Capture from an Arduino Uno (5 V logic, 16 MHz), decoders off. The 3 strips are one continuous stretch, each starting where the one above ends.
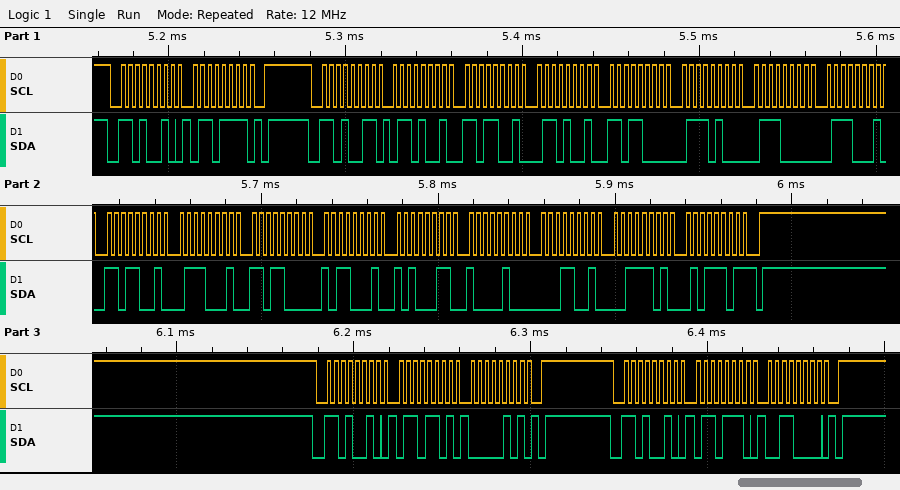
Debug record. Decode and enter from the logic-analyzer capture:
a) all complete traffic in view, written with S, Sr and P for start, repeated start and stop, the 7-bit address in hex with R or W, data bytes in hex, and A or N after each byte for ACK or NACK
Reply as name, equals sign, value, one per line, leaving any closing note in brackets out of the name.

all complete traffic in view, written with S, Sr and P for start, repeated start and stop, the 7-bit address in hex with R or W, data bytes in hex, and A or N after each byte for ACK or NACK = S 69W A 6F A P S 69R A 69 A D9 A 69 A D8 A 74 A 70 A 71 A D9 A 71 A D8 A B1 A A3 A 84 A 19 A 3D A 5D N P S 69W A 6D A 05 A P S 69W A 6E A 30 A P
